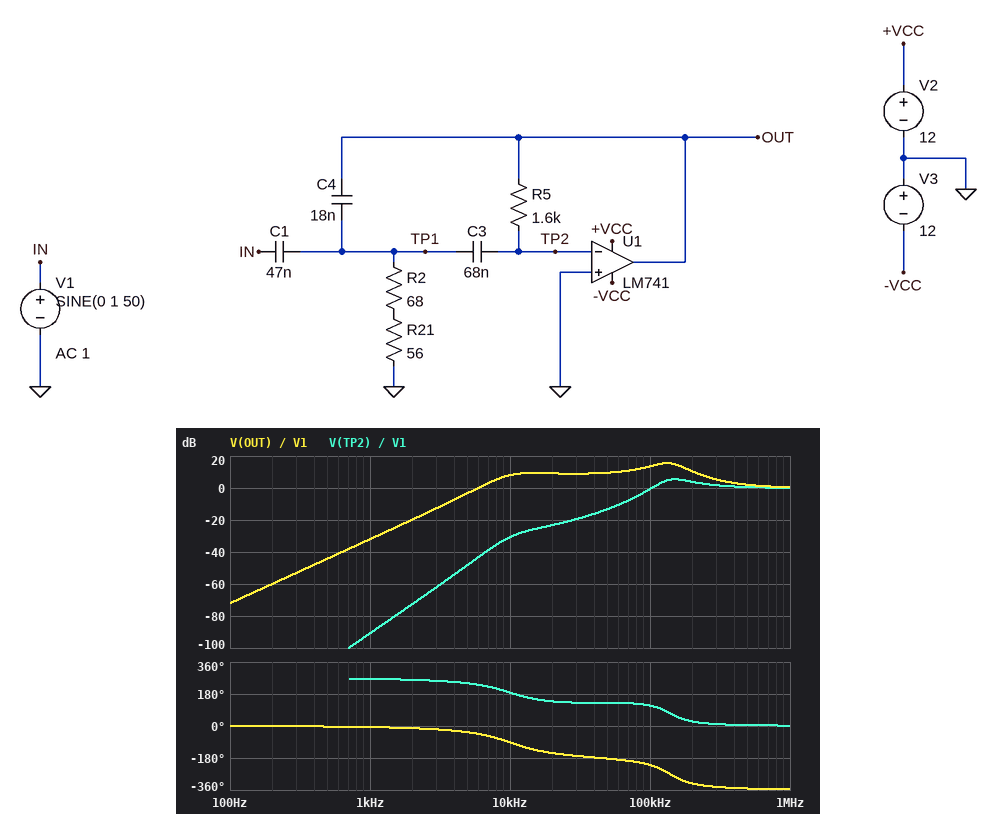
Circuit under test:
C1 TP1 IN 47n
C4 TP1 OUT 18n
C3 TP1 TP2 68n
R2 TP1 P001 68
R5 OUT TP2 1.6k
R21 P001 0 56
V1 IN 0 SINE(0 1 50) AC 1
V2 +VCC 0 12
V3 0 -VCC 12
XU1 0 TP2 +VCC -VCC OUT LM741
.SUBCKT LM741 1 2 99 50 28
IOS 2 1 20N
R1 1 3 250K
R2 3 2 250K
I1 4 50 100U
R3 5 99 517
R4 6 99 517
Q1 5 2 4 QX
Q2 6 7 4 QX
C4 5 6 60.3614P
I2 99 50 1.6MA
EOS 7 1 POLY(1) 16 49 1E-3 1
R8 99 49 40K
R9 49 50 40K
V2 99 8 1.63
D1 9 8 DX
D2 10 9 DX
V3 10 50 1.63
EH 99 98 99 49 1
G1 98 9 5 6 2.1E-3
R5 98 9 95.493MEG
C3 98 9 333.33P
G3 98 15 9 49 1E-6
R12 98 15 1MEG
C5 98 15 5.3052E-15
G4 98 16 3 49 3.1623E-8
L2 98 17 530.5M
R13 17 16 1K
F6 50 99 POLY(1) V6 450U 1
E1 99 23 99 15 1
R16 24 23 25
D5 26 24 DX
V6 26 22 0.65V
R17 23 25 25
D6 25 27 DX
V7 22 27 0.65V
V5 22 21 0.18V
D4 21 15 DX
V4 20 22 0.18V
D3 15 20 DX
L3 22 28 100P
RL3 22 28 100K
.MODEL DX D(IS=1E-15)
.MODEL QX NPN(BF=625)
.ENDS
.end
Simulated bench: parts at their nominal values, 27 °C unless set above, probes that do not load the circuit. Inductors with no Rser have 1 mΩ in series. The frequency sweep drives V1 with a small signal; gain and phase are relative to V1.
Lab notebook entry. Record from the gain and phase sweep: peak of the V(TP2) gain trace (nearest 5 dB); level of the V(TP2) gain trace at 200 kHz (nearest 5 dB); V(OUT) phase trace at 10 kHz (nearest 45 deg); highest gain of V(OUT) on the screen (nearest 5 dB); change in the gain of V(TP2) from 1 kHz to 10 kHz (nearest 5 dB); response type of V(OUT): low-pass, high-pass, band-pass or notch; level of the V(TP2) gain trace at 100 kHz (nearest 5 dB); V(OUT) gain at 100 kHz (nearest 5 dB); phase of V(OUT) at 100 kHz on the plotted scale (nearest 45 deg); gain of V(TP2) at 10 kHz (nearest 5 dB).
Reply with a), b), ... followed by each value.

a) 5 dB
b) 5 dB
c) -90 deg
d) 15 dB
e) 60 dB
f) band-pass
g) 0 dB
h) 15 dB
i) -225 deg
j) -30 dB
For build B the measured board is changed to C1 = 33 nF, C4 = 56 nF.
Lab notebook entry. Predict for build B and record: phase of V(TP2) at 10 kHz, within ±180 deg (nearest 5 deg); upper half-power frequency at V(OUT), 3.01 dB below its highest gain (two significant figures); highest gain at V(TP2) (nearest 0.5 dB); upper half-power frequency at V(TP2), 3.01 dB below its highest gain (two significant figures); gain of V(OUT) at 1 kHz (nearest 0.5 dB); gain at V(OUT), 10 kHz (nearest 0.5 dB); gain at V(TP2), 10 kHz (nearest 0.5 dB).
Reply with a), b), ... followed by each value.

a) 145 deg
b) 210 kHz
c) 8.0 dB
d) 230 kHz
e) -35.0 dB
f) -2.5 dB
g) -40.0 dB
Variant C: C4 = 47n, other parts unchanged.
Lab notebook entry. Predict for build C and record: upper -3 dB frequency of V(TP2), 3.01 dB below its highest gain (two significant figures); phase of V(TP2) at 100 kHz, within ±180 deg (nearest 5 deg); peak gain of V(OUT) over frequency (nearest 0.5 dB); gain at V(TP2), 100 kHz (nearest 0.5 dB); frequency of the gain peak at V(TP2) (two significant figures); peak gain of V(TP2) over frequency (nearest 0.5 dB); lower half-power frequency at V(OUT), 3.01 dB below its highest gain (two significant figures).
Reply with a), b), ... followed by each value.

a) 190 kHz
b) 140 deg
c) 14.0 dB
d) 0 dB
e) 140 kHz
f) 8.5 dB
g) 110 kHz
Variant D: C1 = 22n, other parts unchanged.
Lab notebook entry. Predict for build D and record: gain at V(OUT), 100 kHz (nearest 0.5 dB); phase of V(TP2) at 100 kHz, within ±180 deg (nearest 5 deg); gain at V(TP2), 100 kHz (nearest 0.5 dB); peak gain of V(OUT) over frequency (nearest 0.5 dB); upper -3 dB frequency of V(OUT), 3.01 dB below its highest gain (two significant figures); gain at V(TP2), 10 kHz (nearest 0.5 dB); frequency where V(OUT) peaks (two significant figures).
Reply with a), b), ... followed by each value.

a) 4.5 dB
b) 135 deg
c) -9.5 dB
d) 11.0 dB
e) 280 kHz
f) -35.5 dB
g) 200 kHz
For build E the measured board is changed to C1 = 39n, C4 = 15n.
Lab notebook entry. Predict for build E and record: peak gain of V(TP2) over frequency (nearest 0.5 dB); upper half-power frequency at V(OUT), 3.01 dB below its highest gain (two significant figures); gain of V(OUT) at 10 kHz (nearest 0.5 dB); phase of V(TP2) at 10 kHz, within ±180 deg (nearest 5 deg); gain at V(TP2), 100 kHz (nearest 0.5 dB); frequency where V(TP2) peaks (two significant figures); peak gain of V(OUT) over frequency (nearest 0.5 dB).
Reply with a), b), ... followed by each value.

a) 5.0 dB
b) 200 kHz
c) 7.0 dB
d) -165 deg
e) -3.0 dB
f) 170 kHz
g) 14.5 dB
